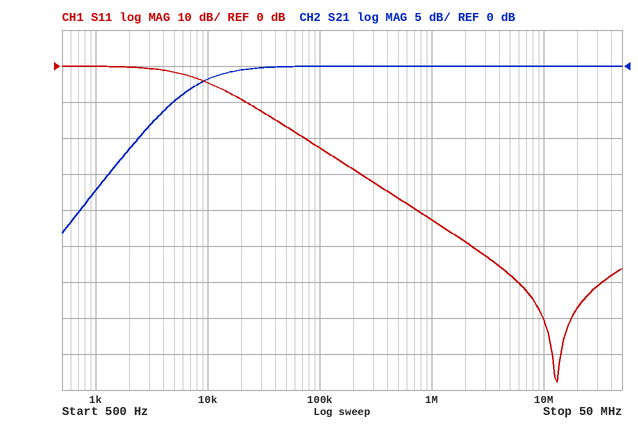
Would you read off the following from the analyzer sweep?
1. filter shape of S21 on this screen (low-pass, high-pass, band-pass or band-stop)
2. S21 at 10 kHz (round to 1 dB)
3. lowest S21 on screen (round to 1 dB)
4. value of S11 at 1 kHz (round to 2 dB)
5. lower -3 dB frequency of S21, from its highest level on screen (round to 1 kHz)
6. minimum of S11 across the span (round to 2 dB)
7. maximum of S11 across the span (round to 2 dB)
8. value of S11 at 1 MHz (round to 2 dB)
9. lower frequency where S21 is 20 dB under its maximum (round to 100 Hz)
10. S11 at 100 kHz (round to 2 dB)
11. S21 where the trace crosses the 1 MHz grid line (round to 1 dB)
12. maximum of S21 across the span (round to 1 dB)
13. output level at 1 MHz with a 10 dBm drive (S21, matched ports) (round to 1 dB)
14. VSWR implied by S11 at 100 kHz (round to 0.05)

high-pass
-2 dB
-23 dB
0 dB
7 kHz
-88 dB
0 dB
-42 dB
700 Hz
-22 dB
0 dB
0 dB
10 dBm
1.15
